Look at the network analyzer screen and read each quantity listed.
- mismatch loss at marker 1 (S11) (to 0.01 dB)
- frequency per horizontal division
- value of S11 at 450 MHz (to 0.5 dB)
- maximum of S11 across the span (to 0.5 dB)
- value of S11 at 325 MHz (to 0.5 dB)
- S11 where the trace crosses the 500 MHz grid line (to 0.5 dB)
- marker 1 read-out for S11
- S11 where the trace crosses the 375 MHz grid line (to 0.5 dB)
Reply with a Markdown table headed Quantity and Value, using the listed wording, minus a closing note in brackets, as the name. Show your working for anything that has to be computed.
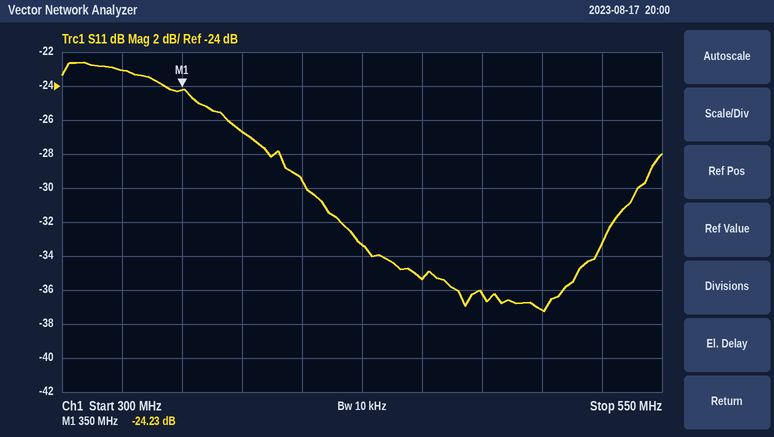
| Quantity | Value |
|---|---|
| mismatch loss at marker 1 (S11) | −10 log10(1 − 10^(-24.23/10)) ≈ 0.02 dB |
| frequency per horizontal division | 25 MHz |
| value of S11 at 450 MHz | -35.5 dB |
| maximum of S11 across the span | -22.5 dB |
| value of S11 at 325 MHz | -23.0 dB |
| S11 where the trace crosses the 500 MHz grid line | -37.0 dB |
| marker 1 read-out for S11 | -24.23 dB |
| S11 where the trace crosses the 375 MHz grid line | -26.5 dB |
